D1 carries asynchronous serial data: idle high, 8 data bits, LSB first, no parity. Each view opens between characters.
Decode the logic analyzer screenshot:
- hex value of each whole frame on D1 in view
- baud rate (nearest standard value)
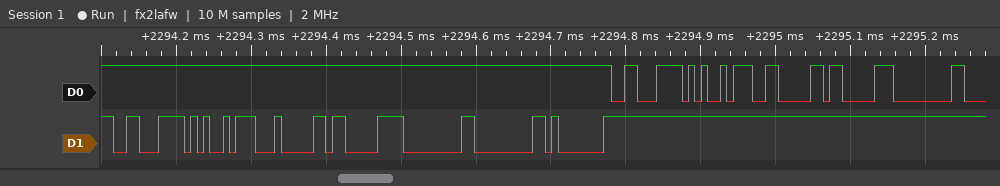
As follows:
C6, A5, 04, 83, 00, 00, 01
115200 baud
